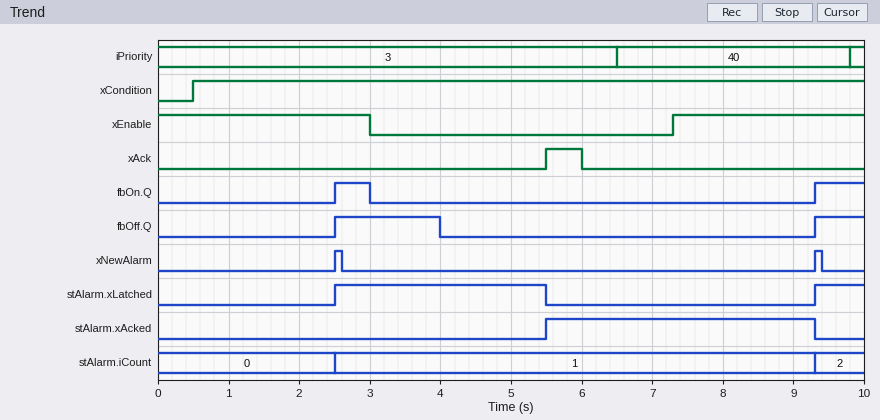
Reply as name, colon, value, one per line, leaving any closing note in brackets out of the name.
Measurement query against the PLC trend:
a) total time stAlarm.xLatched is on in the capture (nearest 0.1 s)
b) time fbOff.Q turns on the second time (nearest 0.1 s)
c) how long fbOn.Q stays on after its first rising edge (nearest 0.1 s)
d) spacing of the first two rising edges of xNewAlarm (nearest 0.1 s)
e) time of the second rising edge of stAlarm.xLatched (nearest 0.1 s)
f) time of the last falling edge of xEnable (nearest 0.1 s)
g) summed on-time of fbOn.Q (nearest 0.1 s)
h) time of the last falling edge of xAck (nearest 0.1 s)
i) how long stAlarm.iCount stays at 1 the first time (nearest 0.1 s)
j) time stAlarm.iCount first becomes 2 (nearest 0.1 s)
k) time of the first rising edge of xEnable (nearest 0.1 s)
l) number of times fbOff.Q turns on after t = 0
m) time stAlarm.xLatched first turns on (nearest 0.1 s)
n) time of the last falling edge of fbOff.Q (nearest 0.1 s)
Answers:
total time stAlarm.xLatched is on in the capture: 3.7 s
time fbOff.Q turns on the second time: 9.3 s
how long fbOn.Q stays on after its first rising edge: 0.5 s
spacing of the first two rising edges of xNewAlarm: 6.8 s
time of the second rising edge of stAlarm.xLatched: 9.3 s
time of the last falling edge of xEnable: 3.0 s
summed on-time of fbOn.Q: 1.2 s
time of the last falling edge of xAck: 6.0 s
how long stAlarm.iCount stays at 1 the first time: 6.8 s
time stAlarm.iCount first becomes 2: 9.3 s
time of the first rising edge of xEnable: 7.3 s
number of times fbOff.Q turns on after t = 0: 2
time stAlarm.xLatched first turns on: 2.5 s
time of the last falling edge of fbOff.Q: 4.0 s
